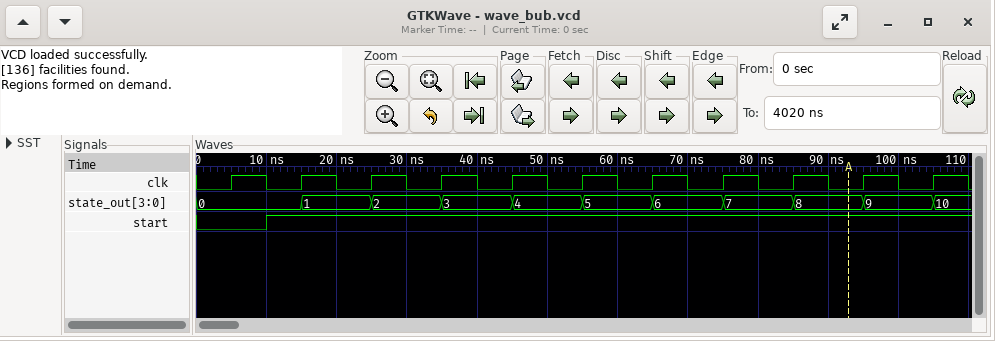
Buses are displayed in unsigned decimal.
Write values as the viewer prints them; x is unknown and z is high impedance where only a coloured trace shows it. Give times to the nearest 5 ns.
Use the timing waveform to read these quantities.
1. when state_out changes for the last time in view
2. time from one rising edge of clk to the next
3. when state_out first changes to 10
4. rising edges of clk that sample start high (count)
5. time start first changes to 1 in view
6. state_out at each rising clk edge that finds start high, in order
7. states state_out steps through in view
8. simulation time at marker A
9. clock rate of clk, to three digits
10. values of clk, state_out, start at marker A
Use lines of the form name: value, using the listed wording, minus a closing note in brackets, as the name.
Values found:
when state_out changes for the last time in view: 105 ns
time from one rising edge of clk to the next: 10 ns
when state_out first changes to 10: 105 ns
rising edges of clk that sample start high: 10
time start first changes to 1 in view: 10 ns
state_out at each rising clk edge that finds start high, in order: 0, 1, 2, 3, 4, 5, 6, 7, 8, 9
states state_out steps through in view: 0, 1, 2, 3, 4, 5, 6, 7, 8, 9, 10
simulation time at marker A: 95 ns
clock rate of clk, to three digits: 100 MHz
values of clk, state_out, start at marker A: clk=0, state_out=8, start=1
